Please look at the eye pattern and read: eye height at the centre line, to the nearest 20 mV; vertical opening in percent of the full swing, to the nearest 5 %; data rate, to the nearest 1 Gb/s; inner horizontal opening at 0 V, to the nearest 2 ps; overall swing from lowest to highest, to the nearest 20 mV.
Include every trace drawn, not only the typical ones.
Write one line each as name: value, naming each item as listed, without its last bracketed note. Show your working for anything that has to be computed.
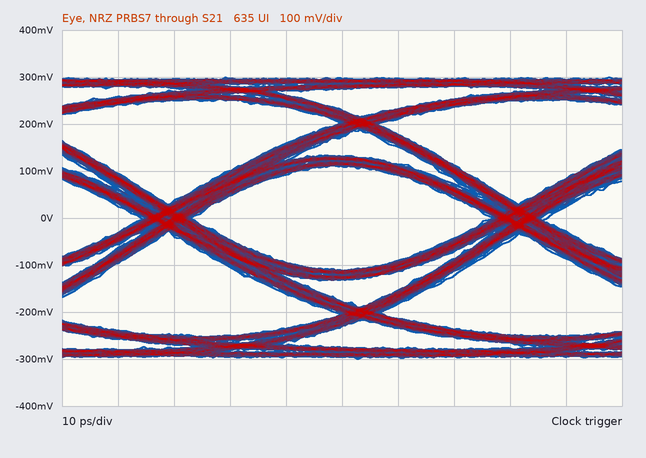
eye height at the centre line, to the nearest 20 mV: 220 mV
vertical opening in percent of the full swing, to the nearest 5 %: 220 mV / 600 mV ≈ 36.7 %, so 35 % to the nearest 5 %
data rate, to the nearest 1 Gb/s: 16 Gb/s
inner horizontal opening at 0 V, to the nearest 2 ps: 54 ps
overall swing from lowest to highest, to the nearest 20 mV: 600 mV
